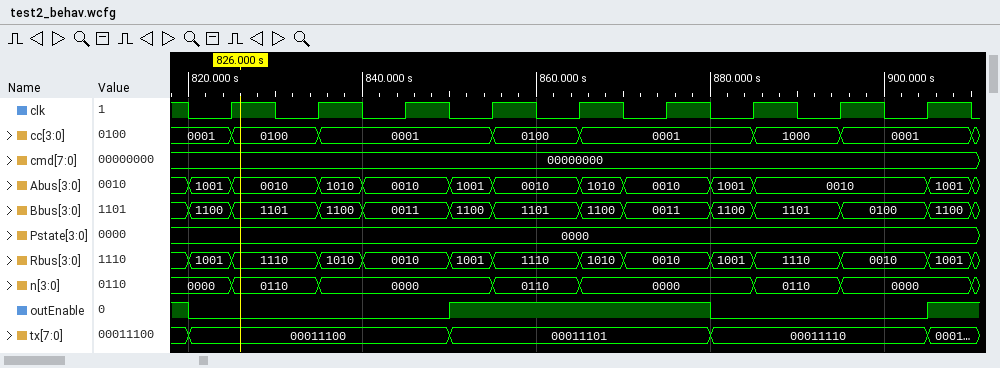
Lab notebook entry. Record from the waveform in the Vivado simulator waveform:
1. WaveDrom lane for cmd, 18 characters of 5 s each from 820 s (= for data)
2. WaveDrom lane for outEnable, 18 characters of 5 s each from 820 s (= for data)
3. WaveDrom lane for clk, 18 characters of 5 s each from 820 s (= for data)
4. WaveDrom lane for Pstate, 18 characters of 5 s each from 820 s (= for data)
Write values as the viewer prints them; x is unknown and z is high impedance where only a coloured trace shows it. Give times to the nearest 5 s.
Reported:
{name: 'cmd', wave: '=.................', data: '00000000'}
{name: 'outEnable', wave: '0.....1.....0....1'}
{name: 'clk', wave: '010101010101010101'}
{name: 'Pstate', wave: '=.................', data: '0000'}
